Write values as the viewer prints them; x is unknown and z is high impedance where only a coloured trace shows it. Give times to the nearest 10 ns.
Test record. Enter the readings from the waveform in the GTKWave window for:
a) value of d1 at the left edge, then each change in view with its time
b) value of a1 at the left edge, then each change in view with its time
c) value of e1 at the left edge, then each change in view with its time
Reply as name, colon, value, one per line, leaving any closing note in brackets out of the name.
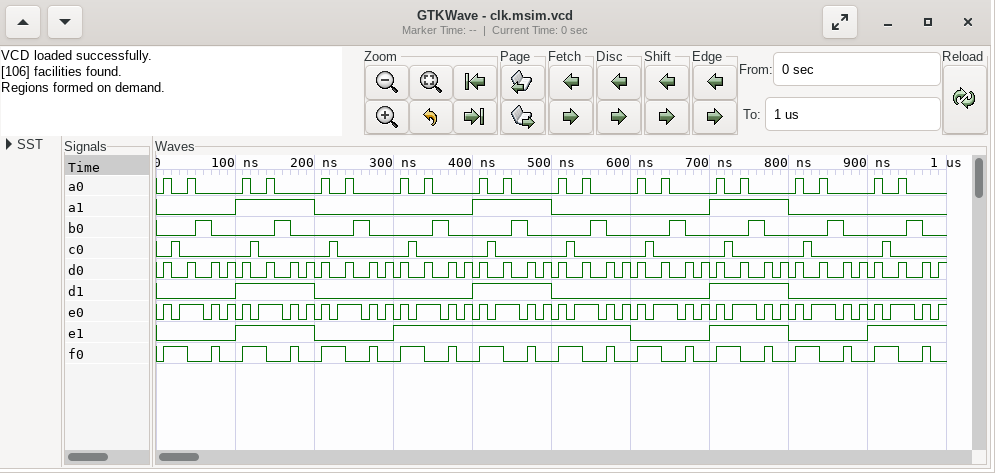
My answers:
value of d1 at the left edge, then each change in view with its time: 0, 1 at 100 ns, 0 at 200 ns, 1 at 400 ns, 0 at 500 ns, 1 at 700 ns, 0 at 800 ns
value of a1 at the left edge, then each change in view with its time: 0, 1 at 100 ns, 0 at 200 ns, 1 at 400 ns, 0 at 500 ns, 1 at 700 ns, 0 at 800 ns
value of e1 at the left edge, then each change in view with its time: 0, 1 at 100 ns, 0 at 200 ns, 1 at 300 ns, 0 at 600 ns, 1 at 700 ns, 0 at 800 ns, 1 at 900 ns
